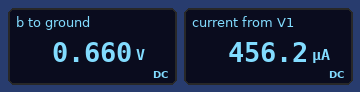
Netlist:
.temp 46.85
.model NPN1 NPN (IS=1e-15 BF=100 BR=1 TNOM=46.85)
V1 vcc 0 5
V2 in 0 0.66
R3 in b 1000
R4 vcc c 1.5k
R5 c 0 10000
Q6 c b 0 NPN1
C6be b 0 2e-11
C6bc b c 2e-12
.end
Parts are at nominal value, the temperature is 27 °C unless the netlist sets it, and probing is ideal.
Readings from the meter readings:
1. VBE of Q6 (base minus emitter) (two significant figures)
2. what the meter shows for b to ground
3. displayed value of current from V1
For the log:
660 mV
0.660 V
456.2 µA
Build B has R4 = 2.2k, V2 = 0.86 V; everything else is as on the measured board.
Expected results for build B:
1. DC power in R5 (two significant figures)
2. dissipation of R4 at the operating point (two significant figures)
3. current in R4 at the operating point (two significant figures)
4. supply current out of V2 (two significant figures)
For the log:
1.1 µW
11 mW
2.2 mA
75 µA
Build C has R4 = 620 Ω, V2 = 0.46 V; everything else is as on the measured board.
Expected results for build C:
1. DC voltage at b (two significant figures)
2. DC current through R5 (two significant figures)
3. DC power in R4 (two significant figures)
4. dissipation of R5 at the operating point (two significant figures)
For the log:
460 mV
470 µA
140 µW
2.2 mW
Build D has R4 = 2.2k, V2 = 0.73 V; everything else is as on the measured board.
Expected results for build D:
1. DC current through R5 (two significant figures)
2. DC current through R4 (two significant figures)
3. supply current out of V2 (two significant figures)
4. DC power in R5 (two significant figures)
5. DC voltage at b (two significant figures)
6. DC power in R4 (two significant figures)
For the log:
360 µA
640 µA
2.8 µA
1.3 mW
730 mV
910 µW
